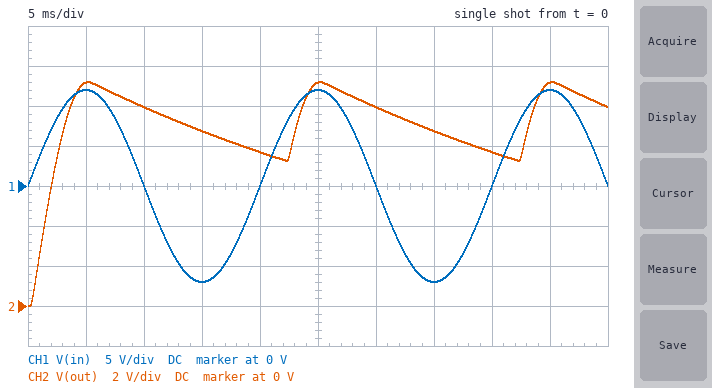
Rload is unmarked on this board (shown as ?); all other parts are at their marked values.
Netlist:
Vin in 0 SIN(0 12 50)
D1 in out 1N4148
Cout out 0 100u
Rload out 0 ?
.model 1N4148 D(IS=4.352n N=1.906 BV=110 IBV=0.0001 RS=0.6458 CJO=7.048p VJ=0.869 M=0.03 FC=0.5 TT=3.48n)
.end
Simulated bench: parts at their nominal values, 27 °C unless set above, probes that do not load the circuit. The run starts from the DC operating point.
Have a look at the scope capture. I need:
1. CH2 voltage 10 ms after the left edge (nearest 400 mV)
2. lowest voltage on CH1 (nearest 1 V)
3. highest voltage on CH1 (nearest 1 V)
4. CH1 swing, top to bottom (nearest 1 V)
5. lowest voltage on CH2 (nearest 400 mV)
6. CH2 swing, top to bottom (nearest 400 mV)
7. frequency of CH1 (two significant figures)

10.0 V
-12 V
12 V
24 V
0 V
11.2 V
50 Hz
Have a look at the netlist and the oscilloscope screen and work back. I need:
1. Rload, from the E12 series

390 Ω
